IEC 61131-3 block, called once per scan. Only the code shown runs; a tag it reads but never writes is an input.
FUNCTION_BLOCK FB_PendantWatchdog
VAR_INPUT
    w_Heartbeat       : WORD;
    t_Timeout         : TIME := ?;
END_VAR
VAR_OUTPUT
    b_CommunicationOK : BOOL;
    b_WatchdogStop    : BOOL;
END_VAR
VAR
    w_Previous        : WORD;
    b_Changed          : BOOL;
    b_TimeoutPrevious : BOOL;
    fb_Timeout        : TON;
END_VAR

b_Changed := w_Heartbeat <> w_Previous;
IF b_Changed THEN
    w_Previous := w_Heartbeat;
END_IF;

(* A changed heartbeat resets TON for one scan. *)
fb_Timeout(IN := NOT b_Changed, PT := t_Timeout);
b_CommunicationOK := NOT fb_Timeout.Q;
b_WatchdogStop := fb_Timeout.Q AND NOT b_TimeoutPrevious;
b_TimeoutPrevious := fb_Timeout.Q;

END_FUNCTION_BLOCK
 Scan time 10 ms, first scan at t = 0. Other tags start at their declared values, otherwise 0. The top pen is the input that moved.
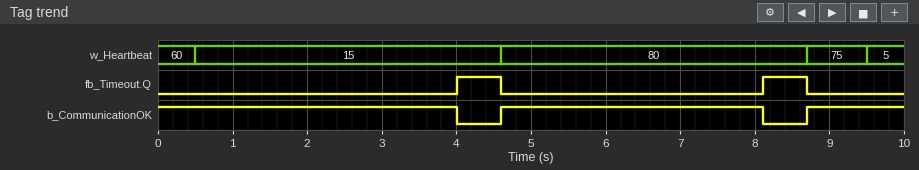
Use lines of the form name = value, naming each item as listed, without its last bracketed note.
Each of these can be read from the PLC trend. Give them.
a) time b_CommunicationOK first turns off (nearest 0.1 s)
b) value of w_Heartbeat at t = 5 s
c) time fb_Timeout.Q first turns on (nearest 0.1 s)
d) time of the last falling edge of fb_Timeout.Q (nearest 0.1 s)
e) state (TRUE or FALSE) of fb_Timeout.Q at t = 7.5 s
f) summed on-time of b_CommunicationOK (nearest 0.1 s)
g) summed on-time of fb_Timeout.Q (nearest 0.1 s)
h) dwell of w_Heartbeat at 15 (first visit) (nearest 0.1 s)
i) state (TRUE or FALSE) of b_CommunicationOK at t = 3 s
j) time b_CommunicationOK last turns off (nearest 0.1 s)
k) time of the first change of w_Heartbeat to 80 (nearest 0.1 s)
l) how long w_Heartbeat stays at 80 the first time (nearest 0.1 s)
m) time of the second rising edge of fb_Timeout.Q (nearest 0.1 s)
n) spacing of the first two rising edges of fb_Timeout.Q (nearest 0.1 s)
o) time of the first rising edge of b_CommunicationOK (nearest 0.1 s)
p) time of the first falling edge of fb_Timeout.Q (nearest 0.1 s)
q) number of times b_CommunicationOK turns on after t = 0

time b_CommunicationOK first turns off = 4.0 s
value of w_Heartbeat at t = 5 s = 80
time fb_Timeout.Q first turns on = 4.0 s
time of the last falling edge of fb_Timeout.Q = 8.7 s
state (TRUE or FALSE) of fb_Timeout.Q at t = 7.5 s = FALSE
summed on-time of b_CommunicationOK = 8.8 s
summed on-time of fb_Timeout.Q = 1.2 s
dwell of w_Heartbeat at 15 (first visit) = 4.1 s
state (TRUE or FALSE) of b_CommunicationOK at t = 3 s = TRUE
time b_CommunicationOK last turns off = 8.1 s
time of the first change of w_Heartbeat to 80 = 4.6 s
how long w_Heartbeat stays at 80 the first time = 4.1 s
time of the second rising edge of fb_Timeout.Q = 8.1 s
spacing of the first two rising edges of fb_Timeout.Q = 4.1 s
time of the first rising edge of b_CommunicationOK = 4.6 s
time of the first falling edge of fb_Timeout.Q = 4.6 s
number of times b_CommunicationOK turns on after t = 0 = 2
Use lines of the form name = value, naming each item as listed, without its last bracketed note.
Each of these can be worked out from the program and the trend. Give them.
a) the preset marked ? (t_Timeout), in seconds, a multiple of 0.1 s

the preset marked ? (t_Timeout), in seconds, a multiple of 0.1 s = 3.5 s
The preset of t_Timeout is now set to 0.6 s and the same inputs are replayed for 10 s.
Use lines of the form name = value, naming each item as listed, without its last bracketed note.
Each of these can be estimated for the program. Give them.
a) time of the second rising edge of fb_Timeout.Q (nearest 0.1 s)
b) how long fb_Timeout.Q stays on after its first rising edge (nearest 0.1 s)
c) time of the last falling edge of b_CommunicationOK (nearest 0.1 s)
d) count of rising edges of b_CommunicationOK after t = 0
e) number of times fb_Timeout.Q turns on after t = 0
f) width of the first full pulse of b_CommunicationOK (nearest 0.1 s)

time of the second rising edge of fb_Timeout.Q = 5.2 s
how long fb_Timeout.Q stays on after its first rising edge = 3.5 s
time of the last falling edge of b_CommunicationOK = 9.3 s
count of rising edges of b_CommunicationOK after t = 0 = 3
number of times fb_Timeout.Q turns on after t = 0 = 3
width of the first full pulse of b_CommunicationOK = 0.6 s
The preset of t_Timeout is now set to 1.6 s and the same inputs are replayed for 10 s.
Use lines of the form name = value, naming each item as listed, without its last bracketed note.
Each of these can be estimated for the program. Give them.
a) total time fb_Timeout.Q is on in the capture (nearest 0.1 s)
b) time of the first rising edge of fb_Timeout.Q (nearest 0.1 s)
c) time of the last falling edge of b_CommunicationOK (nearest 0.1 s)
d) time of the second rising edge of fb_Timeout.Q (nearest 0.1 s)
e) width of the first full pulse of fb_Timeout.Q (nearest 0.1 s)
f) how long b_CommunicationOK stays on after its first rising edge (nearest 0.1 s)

total time fb_Timeout.Q is on in the capture = 5.0 s
time of the first rising edge of fb_Timeout.Q = 2.1 s
time of the last falling edge of b_CommunicationOK = 6.2 s
time of the second rising edge of fb_Timeout.Q = 6.2 s
width of the first full pulse of fb_Timeout.Q = 2.5 s
how long b_CommunicationOK stays on after its first rising edge = 1.6 s
